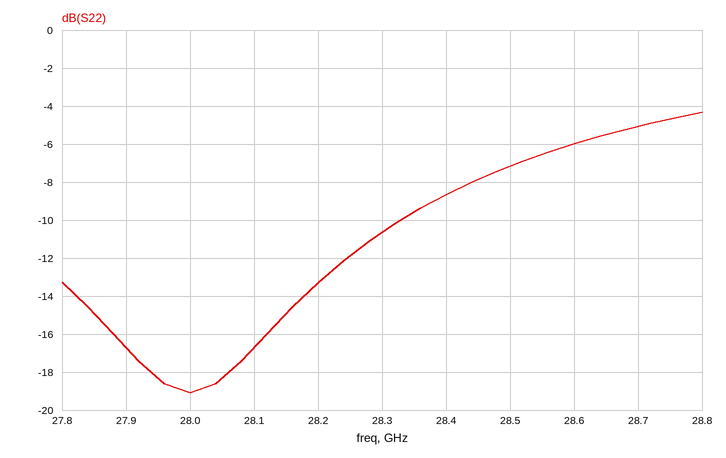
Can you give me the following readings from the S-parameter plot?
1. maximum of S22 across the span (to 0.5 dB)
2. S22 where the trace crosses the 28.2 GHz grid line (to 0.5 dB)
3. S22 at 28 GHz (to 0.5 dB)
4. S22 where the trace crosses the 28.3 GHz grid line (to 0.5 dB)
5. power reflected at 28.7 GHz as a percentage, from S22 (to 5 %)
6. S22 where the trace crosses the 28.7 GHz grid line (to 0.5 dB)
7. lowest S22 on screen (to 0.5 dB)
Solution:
-4.5 dB
-13.5 dB
-19.0 dB
-10.5 dB
30 %
-5.0 dB
-19.0 dB
